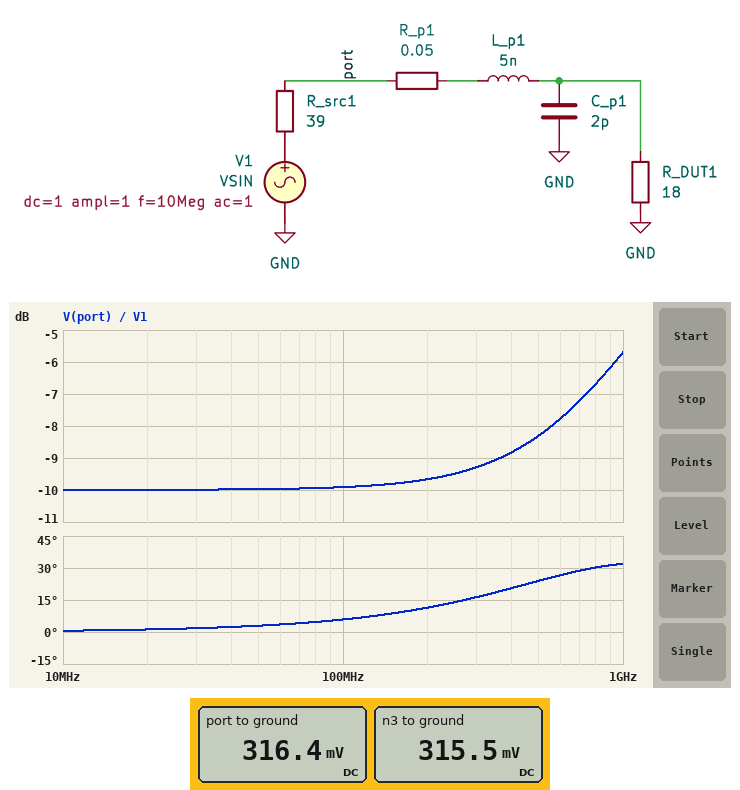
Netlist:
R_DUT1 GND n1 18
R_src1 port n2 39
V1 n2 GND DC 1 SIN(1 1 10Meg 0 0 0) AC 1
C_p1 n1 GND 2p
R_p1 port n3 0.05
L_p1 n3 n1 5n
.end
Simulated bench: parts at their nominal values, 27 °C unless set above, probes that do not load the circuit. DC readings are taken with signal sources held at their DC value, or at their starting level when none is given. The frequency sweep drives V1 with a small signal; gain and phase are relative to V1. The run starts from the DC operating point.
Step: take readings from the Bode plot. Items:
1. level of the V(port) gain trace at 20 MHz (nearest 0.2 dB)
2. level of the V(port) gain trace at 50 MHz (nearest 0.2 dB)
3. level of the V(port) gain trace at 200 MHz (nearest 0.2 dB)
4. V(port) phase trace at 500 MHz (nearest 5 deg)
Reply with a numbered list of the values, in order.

1. -10.0 dB
2. -10.0 dB
3. -9.6 dB
4. 25 deg
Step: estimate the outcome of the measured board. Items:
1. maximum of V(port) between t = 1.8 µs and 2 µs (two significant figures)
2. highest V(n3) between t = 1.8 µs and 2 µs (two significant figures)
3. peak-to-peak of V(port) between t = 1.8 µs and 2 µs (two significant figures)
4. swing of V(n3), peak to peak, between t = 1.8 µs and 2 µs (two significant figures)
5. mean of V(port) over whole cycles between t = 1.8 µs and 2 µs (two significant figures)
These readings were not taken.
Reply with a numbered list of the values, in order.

1. 630 mV
2. 630 mV
3. 630 mV
4. 630 mV
5. 320 mV
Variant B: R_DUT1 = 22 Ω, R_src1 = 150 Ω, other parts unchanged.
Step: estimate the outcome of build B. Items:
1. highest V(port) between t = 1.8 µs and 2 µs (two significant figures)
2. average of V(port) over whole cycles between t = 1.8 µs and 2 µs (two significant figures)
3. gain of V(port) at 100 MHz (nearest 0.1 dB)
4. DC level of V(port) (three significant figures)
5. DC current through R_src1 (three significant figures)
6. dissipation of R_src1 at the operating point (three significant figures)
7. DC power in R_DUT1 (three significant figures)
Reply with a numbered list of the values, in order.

1. 260 mV
2. 130 mV
3. -17.8 dB
4. 128 mV
5. 5.81 mA
6. 5.07 mW
7. 743 µW
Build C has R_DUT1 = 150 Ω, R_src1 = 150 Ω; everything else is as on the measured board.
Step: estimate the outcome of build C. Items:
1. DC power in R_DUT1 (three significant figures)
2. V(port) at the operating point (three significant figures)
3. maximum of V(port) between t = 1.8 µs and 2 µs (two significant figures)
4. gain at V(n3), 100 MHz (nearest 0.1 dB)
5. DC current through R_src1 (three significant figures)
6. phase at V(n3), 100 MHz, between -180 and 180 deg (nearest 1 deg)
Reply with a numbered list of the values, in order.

1. 1.67 mW
2. 500 mV
3. 1.0 V
4. -6.1 dB
5. 3.33 mA
6. -5 deg
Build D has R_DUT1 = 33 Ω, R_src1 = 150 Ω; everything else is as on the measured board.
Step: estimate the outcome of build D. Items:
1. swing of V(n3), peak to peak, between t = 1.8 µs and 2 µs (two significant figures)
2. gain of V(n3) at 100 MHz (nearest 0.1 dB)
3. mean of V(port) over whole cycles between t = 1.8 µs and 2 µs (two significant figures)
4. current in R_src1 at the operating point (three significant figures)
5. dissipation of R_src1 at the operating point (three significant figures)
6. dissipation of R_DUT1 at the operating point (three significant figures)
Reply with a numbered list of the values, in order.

1. 360 mV
2. -14.9 dB
3. 180 mV
4. 5.46 mA
5. 4.48 mW
6. 985 µW
